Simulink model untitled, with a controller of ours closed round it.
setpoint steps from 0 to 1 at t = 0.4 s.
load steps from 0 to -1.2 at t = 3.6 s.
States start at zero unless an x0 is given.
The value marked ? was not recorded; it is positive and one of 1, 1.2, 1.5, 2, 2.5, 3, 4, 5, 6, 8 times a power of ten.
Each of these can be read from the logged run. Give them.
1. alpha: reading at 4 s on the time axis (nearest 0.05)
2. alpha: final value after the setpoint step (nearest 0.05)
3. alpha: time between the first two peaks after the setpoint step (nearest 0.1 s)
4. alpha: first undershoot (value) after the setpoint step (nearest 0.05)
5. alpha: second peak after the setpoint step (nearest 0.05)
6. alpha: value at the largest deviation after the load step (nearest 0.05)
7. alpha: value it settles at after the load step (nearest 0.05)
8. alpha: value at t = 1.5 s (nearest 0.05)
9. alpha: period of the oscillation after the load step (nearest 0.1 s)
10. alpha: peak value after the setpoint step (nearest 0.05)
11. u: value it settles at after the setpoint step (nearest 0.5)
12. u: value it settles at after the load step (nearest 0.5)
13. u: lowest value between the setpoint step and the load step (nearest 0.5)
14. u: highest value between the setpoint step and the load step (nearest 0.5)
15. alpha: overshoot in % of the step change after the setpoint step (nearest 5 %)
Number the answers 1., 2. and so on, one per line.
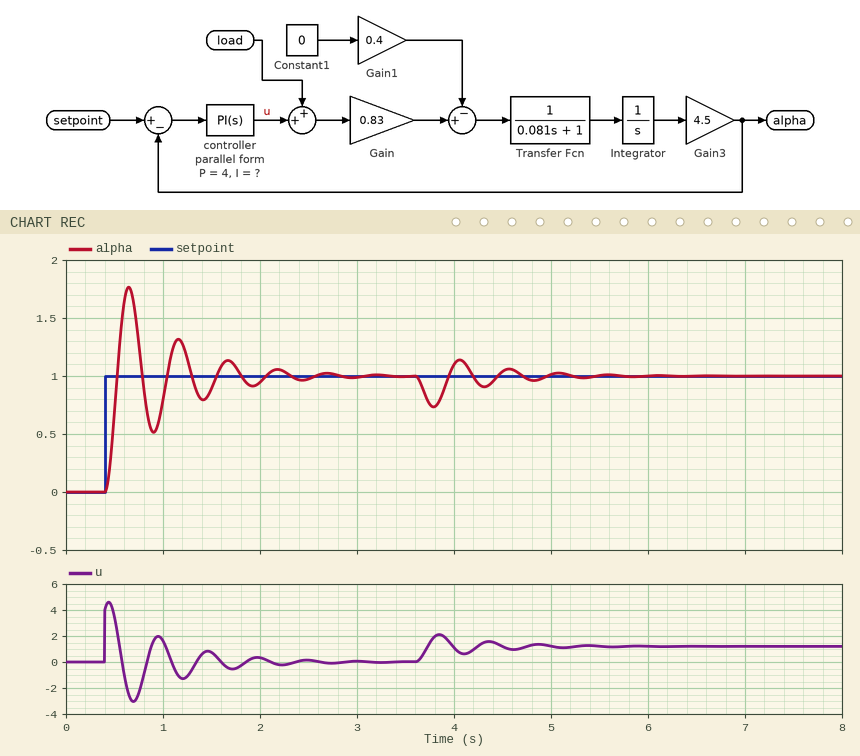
1. 1.10
2. 1.00
3. 0.5 s
4. 0.50
5. 1.30
6. 0.75
7. 1.00
8. 0.90
9. 0.5 s
10. 1.75
11. 0.0
12. 1.0
13. -3.0
14. 4.5
15. 75 %
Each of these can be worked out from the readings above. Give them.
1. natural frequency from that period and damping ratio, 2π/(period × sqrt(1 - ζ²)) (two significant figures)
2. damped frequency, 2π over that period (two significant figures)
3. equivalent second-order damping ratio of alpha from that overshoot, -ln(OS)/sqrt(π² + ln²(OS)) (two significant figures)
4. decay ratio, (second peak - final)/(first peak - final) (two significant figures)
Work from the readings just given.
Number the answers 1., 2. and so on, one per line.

1. 13 rad/s
2. 13 rad/s
3. 0.091
4. 0.40
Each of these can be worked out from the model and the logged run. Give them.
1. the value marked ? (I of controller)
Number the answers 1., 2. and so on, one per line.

1. 30
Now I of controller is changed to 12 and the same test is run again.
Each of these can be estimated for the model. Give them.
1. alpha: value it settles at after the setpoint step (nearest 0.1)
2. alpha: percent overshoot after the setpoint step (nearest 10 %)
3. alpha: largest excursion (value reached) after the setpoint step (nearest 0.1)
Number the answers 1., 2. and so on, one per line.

1. 1.0
2. 50 %
3. 1.5
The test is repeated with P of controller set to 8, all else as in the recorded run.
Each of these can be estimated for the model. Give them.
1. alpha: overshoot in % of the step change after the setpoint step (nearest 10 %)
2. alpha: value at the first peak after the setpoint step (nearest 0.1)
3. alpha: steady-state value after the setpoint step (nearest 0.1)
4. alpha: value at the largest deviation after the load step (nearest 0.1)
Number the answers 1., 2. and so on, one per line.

1. 60 %
2. 1.6
3. 1.0
4. 0.8
